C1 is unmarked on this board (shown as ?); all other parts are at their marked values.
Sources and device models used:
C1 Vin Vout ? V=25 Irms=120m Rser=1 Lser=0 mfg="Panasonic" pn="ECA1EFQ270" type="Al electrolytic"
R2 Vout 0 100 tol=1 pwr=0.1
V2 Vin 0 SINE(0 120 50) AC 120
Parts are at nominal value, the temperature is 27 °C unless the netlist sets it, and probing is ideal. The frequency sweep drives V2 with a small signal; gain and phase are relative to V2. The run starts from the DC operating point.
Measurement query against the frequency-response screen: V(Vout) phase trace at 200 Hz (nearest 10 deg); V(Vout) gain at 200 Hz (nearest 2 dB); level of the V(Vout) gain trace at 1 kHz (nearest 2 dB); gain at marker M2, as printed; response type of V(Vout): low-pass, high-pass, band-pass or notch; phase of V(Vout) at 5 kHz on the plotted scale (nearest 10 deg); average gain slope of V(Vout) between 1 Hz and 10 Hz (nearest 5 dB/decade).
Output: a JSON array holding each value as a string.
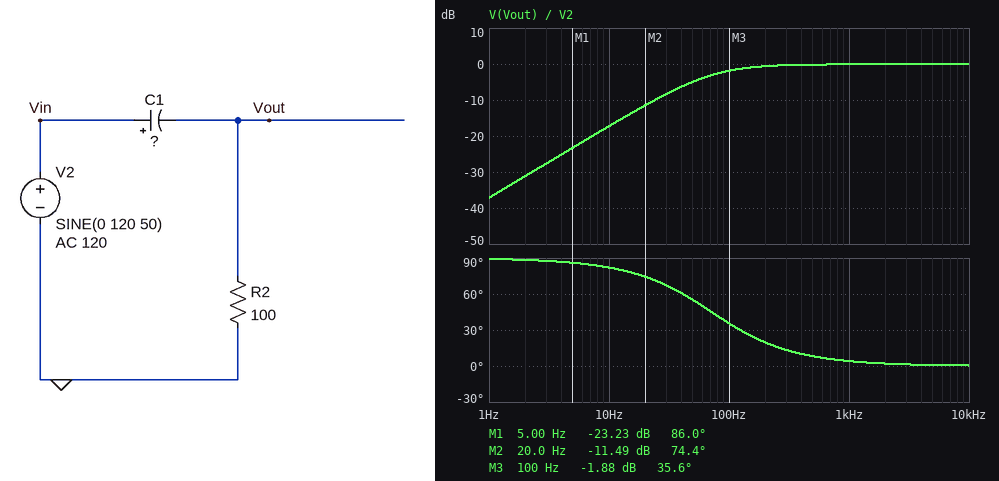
["20 deg", "0 dB", "0 dB", "-11.49 dB", "high-pass", "0 deg", "20 dB/decade"]
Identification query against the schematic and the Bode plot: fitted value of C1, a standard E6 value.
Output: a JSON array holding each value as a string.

["22 µF"]
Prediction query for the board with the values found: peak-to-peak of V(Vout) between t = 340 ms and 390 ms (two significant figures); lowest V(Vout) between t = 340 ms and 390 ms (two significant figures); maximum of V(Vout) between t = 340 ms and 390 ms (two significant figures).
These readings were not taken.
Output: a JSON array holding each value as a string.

["140 V", "-68 V", "68 V"]
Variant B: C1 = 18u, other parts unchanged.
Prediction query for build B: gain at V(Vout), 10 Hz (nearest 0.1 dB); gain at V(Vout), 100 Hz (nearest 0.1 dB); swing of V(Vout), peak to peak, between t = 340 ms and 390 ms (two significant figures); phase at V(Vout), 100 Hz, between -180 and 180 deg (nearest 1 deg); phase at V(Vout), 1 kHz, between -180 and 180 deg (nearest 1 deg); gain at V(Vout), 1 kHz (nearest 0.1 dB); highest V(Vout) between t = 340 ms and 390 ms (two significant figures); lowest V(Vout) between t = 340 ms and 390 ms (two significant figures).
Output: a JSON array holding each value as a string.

["-19.0 dB", "-2.6 dB", "120 V", "41 deg", "5 deg", "-0.1 dB", "59 V", "-59 V"]
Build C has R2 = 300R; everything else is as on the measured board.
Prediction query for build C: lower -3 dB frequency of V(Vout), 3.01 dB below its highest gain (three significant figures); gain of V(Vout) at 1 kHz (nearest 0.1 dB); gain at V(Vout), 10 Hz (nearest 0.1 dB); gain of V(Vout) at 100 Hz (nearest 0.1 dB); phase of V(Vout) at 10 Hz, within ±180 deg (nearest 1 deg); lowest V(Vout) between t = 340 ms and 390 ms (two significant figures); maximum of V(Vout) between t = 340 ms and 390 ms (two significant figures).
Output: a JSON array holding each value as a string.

["24.0 Hz", "0 dB", "-8.3 dB", "-0.3 dB", "67 deg", "-110 V", "110 V"]
